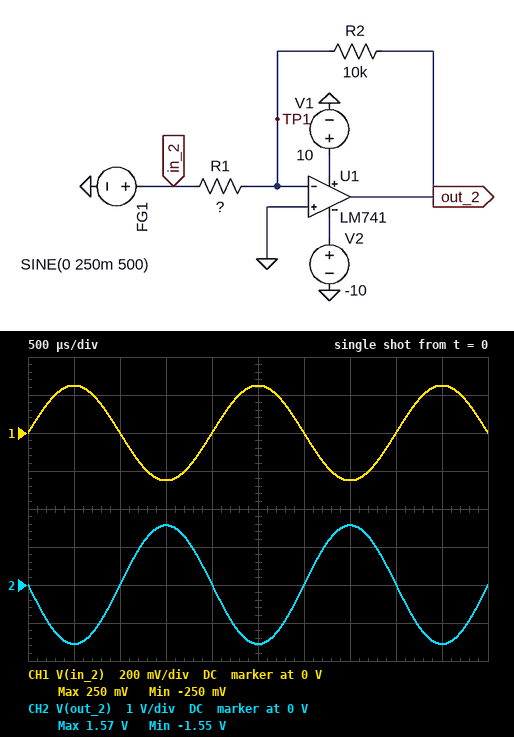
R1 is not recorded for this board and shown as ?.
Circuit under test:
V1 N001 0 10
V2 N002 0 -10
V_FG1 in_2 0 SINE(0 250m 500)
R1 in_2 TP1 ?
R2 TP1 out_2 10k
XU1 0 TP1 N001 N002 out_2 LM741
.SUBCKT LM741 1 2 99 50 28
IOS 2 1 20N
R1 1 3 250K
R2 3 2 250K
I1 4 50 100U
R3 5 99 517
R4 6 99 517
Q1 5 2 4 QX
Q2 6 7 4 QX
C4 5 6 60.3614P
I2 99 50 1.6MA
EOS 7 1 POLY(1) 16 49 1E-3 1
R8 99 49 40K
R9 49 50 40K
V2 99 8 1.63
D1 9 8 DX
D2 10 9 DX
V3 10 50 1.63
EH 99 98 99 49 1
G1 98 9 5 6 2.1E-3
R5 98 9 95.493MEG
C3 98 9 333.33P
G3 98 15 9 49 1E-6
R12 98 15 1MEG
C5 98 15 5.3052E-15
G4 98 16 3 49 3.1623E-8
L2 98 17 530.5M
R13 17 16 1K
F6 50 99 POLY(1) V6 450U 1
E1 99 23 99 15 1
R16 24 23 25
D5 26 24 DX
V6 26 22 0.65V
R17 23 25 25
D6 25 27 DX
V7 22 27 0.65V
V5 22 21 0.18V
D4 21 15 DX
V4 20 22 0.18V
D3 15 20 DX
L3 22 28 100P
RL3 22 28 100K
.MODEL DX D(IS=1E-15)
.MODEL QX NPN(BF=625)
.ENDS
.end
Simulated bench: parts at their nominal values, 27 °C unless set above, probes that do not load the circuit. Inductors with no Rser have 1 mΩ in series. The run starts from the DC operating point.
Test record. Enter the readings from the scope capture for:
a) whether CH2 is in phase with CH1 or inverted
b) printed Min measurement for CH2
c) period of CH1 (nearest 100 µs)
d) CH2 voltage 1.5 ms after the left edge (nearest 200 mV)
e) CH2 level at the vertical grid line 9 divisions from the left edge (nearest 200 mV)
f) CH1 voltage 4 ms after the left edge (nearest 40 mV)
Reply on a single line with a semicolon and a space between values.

inverted; -1.55 V; 2.0 ms; 1.6 V; -1.6 V; 0 V
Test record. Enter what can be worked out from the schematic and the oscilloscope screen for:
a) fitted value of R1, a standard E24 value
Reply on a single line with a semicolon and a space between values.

1.6 kΩ
